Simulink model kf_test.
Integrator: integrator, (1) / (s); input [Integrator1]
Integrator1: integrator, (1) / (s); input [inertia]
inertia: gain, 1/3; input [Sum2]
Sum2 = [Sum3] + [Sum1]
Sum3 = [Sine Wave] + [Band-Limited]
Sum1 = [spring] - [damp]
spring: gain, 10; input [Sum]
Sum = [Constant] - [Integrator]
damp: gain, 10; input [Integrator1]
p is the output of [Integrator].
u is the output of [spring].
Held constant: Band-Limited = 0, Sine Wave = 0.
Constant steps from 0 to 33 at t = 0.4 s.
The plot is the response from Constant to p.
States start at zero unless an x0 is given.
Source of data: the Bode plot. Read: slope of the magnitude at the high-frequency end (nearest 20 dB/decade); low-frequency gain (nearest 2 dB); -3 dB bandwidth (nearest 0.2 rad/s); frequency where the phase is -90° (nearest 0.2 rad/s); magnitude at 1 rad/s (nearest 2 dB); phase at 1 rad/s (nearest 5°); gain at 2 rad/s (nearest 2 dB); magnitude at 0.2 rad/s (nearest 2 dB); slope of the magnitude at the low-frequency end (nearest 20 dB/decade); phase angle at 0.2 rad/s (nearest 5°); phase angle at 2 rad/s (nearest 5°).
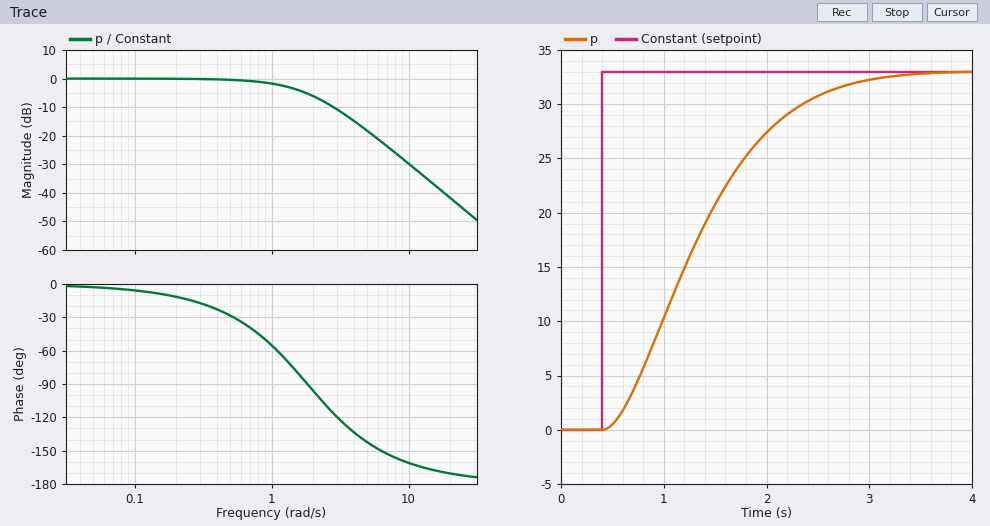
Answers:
-40 dB/decade
0 dB
1.4 rad/s
1.8 rad/s
-2 dB
-55°
-6 dB
0 dB
0 dB/decade
-10°
-95°
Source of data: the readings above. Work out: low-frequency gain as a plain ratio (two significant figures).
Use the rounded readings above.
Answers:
1.0
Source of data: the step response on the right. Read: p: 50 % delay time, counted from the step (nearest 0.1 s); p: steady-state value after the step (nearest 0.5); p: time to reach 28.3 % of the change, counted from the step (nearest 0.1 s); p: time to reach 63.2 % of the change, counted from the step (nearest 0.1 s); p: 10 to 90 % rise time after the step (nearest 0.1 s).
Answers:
0.9 s
33.0
0.6 s
1.1 s
1.6 s
